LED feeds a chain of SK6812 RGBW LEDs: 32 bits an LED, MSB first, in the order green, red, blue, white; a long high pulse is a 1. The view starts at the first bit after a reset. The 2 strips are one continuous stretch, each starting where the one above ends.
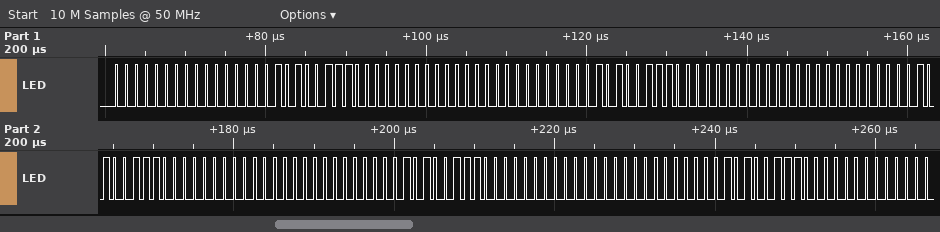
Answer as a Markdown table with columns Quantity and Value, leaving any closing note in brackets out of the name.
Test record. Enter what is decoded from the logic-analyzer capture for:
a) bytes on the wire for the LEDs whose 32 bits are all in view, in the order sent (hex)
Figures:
| Quantity | Value |
|---|---|
| bytes on the wire for the LEDs whose 32 bits are all in view, in the order sent | 00 00 A7 00 00 00 A7 00 00 00 A7 00 00 00 A7 00 00 00 A7 00 |
